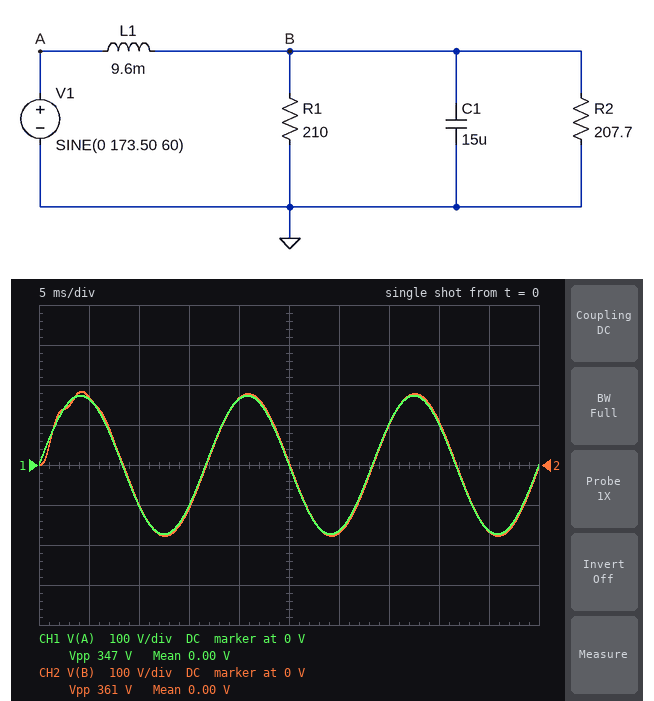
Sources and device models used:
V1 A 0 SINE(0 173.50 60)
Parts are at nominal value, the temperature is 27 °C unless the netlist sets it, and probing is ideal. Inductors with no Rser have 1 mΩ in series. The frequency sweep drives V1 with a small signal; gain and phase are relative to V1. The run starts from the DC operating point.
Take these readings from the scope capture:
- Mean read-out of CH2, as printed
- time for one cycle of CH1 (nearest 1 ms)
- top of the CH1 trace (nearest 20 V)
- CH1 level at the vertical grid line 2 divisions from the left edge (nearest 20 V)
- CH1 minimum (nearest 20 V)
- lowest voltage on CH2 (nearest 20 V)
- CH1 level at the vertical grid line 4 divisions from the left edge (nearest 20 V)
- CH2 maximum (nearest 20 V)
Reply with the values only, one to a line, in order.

0.00 V
17 ms
180 V
-100 V
-180 V
-180 V
160 V
180 V
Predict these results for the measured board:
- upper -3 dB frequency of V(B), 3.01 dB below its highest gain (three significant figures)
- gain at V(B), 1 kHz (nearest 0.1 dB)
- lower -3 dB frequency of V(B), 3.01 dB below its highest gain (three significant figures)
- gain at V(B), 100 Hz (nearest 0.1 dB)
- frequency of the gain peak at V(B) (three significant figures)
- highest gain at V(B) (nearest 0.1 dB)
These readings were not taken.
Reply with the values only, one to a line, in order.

462 Hz
-13.5 dB
358 Hz
0.5 dB
413 Hz
12.4 dB
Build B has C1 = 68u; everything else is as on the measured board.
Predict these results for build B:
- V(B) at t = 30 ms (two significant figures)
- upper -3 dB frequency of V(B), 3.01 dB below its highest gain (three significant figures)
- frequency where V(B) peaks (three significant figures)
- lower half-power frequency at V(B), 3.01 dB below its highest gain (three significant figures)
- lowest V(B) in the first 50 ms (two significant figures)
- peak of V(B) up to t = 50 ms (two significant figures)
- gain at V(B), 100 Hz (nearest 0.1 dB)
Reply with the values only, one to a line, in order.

-180 V
207 Hz
196 Hz
185 Hz
-210 V
230 V
2.6 dB
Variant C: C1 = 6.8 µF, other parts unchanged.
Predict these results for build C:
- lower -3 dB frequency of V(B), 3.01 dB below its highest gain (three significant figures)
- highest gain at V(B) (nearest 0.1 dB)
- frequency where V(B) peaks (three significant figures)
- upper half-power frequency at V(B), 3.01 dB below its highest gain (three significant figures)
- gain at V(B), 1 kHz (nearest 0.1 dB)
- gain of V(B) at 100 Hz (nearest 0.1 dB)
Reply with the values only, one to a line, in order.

475 Hz
9.0 dB
602 Hz
707 Hz
-4.5 dB
0.2 dB
